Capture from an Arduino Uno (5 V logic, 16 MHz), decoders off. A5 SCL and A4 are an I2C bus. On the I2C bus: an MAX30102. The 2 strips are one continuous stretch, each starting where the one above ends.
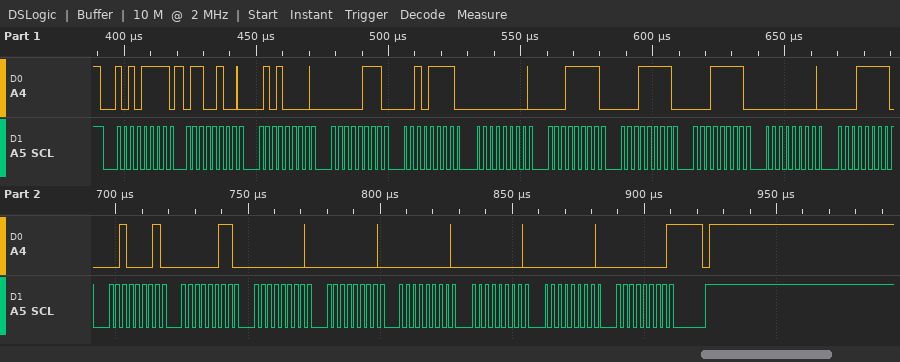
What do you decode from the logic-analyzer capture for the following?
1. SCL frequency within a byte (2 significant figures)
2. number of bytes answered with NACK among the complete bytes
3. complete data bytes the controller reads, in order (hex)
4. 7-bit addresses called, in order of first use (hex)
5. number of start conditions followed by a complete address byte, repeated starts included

400 kHz
1
64 50 07 2F 00 1F 1F 1F 00 1F 21 03 00 00 00 00 00 00
0x57
1
